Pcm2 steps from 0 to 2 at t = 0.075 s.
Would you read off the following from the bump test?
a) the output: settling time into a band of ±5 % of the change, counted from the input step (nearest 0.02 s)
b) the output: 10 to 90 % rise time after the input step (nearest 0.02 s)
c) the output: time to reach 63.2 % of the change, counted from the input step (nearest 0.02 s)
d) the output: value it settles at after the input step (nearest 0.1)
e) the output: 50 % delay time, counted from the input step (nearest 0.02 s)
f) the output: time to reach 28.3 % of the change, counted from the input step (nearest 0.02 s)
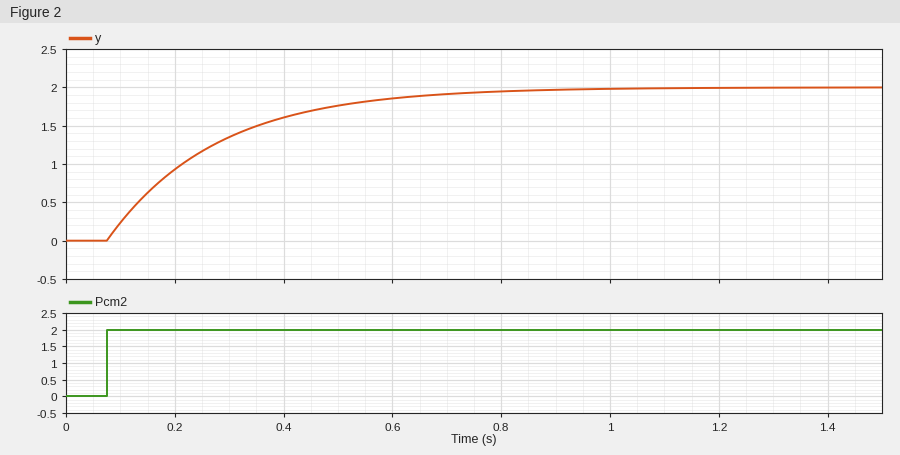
0.60 s
0.44 s
0.20 s
2.0
0.14 s
0.06 s
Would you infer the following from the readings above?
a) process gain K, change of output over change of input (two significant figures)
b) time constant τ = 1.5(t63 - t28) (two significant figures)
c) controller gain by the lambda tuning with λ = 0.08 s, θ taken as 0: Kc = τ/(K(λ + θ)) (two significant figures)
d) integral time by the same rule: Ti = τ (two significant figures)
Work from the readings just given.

1.0
0.21 s
2.6
0.21 s
